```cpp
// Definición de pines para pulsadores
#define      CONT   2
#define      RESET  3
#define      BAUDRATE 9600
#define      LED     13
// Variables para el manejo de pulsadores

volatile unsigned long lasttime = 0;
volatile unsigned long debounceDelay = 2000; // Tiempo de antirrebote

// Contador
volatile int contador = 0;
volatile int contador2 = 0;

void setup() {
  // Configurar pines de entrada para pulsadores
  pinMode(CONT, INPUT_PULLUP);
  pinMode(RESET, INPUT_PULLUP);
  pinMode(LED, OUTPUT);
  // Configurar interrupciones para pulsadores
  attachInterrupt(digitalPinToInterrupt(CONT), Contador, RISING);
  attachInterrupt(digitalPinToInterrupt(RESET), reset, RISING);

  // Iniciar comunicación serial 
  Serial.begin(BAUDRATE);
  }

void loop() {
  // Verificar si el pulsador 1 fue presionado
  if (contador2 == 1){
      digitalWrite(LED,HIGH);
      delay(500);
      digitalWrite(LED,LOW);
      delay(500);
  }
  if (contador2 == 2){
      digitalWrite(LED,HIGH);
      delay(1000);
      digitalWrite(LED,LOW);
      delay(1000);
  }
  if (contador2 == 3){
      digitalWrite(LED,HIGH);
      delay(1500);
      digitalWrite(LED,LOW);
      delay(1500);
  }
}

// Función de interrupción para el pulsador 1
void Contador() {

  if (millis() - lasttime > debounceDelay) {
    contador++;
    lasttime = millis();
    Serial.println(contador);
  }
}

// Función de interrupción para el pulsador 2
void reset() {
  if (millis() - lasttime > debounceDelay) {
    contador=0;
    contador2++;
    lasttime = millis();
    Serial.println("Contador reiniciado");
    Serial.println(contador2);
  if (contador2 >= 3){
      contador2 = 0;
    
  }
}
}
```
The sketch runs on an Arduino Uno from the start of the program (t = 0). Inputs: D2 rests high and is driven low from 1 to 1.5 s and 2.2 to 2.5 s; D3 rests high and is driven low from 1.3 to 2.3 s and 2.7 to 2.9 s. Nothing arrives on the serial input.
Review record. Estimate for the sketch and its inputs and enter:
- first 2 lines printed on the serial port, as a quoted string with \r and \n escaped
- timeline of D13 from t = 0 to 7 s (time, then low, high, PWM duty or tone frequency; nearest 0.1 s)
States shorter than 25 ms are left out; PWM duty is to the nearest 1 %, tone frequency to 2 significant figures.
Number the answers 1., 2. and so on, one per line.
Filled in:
1. "Contador reiniciado\r\n1\r\n"
2. 0 s low; 2.3 s high; 2.8 s low; 3.3 s high; 3.8 s low; 4.3 s high; 4.8 s low; 5.3 s high; 5.8 s low; 6.3 s high; 6.8 s low
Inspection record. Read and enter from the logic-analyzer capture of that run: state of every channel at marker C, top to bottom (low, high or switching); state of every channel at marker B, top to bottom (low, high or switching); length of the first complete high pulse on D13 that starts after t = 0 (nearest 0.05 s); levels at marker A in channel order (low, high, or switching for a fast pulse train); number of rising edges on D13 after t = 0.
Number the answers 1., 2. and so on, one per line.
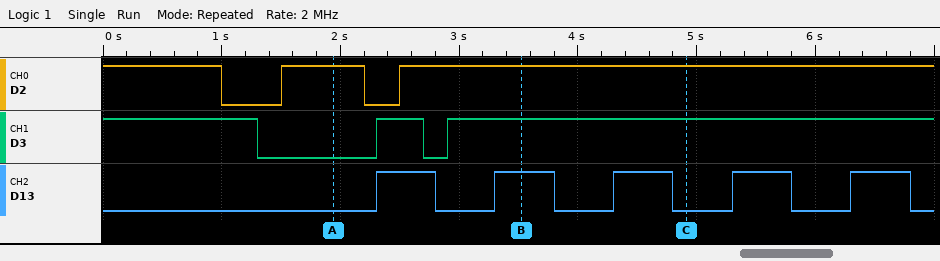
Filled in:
1. D2 high, D3 high, D13 low
2. D2 high, D3 high, D13 high
3. 0.50 s
4. D2 high, D3 low, D13 low
5. 5
